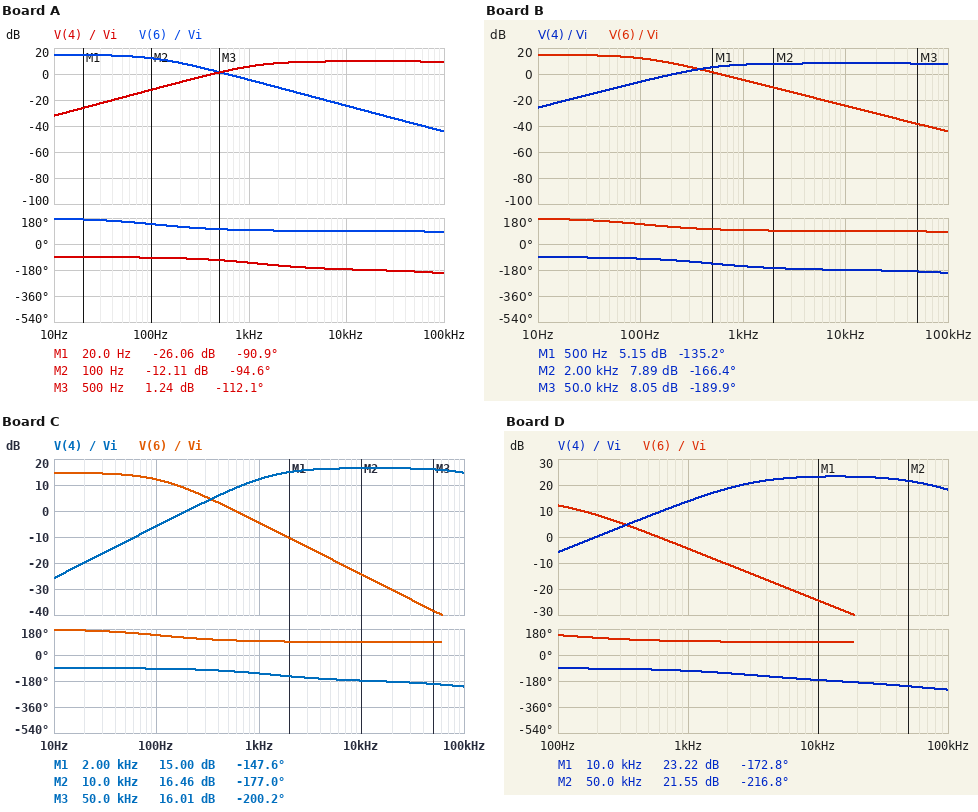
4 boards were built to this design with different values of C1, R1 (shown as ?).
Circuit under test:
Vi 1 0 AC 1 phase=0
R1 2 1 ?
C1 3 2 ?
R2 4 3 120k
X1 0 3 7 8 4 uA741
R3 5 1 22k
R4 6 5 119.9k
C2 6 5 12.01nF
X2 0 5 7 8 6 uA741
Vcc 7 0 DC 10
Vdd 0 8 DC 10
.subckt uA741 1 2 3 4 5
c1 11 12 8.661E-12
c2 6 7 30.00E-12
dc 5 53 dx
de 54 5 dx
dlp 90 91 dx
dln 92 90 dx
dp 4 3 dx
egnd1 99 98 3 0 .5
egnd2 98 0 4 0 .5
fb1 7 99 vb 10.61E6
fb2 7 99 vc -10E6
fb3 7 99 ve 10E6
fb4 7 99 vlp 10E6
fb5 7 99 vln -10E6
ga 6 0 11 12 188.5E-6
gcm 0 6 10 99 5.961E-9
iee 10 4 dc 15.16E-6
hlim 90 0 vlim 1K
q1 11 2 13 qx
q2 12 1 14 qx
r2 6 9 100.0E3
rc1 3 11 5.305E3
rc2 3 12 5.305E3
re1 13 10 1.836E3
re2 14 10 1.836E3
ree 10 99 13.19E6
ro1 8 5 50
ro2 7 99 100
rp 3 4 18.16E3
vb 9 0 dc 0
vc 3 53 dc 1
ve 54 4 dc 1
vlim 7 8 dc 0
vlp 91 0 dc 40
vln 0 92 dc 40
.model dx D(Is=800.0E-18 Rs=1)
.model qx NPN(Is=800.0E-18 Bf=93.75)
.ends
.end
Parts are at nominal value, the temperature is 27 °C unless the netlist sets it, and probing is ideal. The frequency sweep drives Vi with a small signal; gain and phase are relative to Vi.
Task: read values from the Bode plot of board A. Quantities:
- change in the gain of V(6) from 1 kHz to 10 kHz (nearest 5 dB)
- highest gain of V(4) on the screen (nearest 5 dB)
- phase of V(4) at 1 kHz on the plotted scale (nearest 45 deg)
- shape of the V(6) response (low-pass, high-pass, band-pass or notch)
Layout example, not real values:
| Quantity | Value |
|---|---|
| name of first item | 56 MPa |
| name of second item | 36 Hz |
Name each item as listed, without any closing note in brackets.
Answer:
| Quantity | Value |
|---|---|
| change in the gain of V(6) from 1 kHz to 10 kHz | -20 dB |
| highest gain of V(4) on the screen | 10 dB |
| phase of V(4) at 1 kHz on the plotted scale | -135 deg |
| shape of the V(6) response | low-pass |
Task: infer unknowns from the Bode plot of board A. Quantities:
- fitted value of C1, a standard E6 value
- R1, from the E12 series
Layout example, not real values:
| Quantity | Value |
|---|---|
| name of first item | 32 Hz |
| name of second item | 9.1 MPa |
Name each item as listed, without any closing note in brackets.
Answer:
| Quantity | Value |
|---|---|
| fitted value of C1, a standard E6 value | 3.3 nF |
| R1, from the E12 series | 39 kΩ |
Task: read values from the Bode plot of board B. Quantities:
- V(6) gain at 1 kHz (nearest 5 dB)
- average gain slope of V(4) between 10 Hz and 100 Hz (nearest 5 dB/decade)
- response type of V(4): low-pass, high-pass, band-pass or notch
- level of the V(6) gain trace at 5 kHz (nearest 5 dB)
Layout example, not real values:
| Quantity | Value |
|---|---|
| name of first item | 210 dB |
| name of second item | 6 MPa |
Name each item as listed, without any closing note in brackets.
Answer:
| Quantity | Value |
|---|---|
| V(6) gain at 1 kHz | -5 dB |
| average gain slope of V(4) between 10 Hz and 100 Hz | 20 dB/decade |
| response type of V(4): low-pass, high-pass, band-pass or notch | high-pass |
| level of the V(6) gain trace at 5 kHz | -20 dB |
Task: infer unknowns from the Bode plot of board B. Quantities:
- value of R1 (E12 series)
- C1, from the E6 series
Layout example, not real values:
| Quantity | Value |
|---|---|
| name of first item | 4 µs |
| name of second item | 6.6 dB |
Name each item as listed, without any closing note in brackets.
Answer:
| Quantity | Value |
|---|---|
| value of R1 | 47 kΩ |
| C1, from the E6 series | 6.8 nF |
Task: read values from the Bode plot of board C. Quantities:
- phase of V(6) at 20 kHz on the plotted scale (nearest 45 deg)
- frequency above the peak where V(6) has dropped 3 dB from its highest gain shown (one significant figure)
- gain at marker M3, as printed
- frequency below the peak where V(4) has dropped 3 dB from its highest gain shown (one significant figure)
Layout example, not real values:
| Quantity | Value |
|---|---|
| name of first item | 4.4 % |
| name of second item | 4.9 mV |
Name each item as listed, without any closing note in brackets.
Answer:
| Quantity | Value |
|---|---|
| phase of V(6) at 20 kHz on the plotted scale | 90 deg |
| frequency above the peak where V(6) has dropped 3 dB from its highest gain shown | 100 Hz |
| gain at marker M3, as printed | 16.01 dB |
| frequency below the peak where V(4) has dropped 3 dB from its highest gain shown | 1 kHz |
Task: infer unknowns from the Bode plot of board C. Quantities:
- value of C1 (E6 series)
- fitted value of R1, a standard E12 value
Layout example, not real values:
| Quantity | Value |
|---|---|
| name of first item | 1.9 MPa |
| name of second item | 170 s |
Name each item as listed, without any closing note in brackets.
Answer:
| Quantity | Value |
|---|---|
| value of C1 | 6.8 nF |
| fitted value of R1, a standard E12 value | 18 kΩ |
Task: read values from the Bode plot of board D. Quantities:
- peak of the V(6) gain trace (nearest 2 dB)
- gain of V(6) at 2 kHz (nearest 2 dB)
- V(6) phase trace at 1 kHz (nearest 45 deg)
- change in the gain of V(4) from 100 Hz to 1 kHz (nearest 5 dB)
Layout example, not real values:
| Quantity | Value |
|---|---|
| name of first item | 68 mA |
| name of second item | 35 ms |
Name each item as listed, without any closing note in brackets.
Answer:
| Quantity | Value |
|---|---|
| peak of the V(6) gain trace | 12 dB |
| gain of V(6) at 2 kHz | -10 dB |
| V(6) phase trace at 1 kHz | 90 deg |
| change in the gain of V(4) from 100 Hz to 1 kHz | 20 dB |
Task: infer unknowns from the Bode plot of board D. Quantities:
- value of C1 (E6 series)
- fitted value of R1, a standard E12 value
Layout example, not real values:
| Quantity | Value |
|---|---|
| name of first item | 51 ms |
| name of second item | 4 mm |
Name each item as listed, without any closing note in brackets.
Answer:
| Quantity | Value |
|---|---|
| value of C1 | 6.8 nF |
| fitted value of R1, a standard E12 value | 8.2 kΩ |
